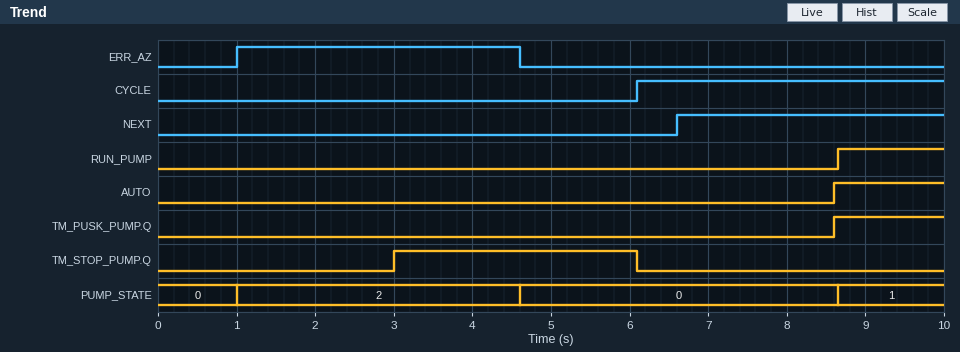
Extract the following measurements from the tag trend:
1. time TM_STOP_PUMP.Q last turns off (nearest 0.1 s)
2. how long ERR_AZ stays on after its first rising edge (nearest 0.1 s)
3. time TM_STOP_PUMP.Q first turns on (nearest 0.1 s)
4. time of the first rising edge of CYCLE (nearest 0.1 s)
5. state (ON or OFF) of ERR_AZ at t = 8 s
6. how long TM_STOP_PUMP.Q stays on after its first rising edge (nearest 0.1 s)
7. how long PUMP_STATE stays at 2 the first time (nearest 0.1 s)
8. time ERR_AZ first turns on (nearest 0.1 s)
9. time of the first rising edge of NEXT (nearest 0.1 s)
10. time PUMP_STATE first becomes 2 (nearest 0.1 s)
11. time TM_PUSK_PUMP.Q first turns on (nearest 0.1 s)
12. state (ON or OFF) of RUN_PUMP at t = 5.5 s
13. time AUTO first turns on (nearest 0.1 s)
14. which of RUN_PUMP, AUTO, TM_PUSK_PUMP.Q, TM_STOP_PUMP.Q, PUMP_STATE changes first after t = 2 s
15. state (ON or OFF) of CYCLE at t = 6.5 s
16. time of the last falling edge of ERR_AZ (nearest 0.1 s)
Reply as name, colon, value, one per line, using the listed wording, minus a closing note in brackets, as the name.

time TM_STOP_PUMP.Q last turns off: 6.1 s
how long ERR_AZ stays on after its first rising edge: 3.6 s
time TM_STOP_PUMP.Q first turns on: 3.0 s
time of the first rising edge of CYCLE: 6.1 s
state (ON or OFF) of ERR_AZ at t = 8 s: OFF
how long TM_STOP_PUMP.Q stays on after its first rising edge: 3.1 s
how long PUMP_STATE stays at 2 the first time: 3.6 s
time ERR_AZ first turns on: 1.0 s
time of the first rising edge of NEXT: 6.6 s
time PUMP_STATE first becomes 2: 1.0 s
time TM_PUSK_PUMP.Q first turns on: 8.6 s
state (ON or OFF) of RUN_PUMP at t = 5.5 s: OFF
time AUTO first turns on: 8.6 s
which of RUN_PUMP, AUTO, TM_PUSK_PUMP.Q, TM_STOP_PUMP.Q, PUMP_STATE changes first after t = 2 s: TM_STOP_PUMP.Q
state (ON or OFF) of CYCLE at t = 6.5 s: ON
time of the last falling edge of ERR_AZ: 4.6 s
